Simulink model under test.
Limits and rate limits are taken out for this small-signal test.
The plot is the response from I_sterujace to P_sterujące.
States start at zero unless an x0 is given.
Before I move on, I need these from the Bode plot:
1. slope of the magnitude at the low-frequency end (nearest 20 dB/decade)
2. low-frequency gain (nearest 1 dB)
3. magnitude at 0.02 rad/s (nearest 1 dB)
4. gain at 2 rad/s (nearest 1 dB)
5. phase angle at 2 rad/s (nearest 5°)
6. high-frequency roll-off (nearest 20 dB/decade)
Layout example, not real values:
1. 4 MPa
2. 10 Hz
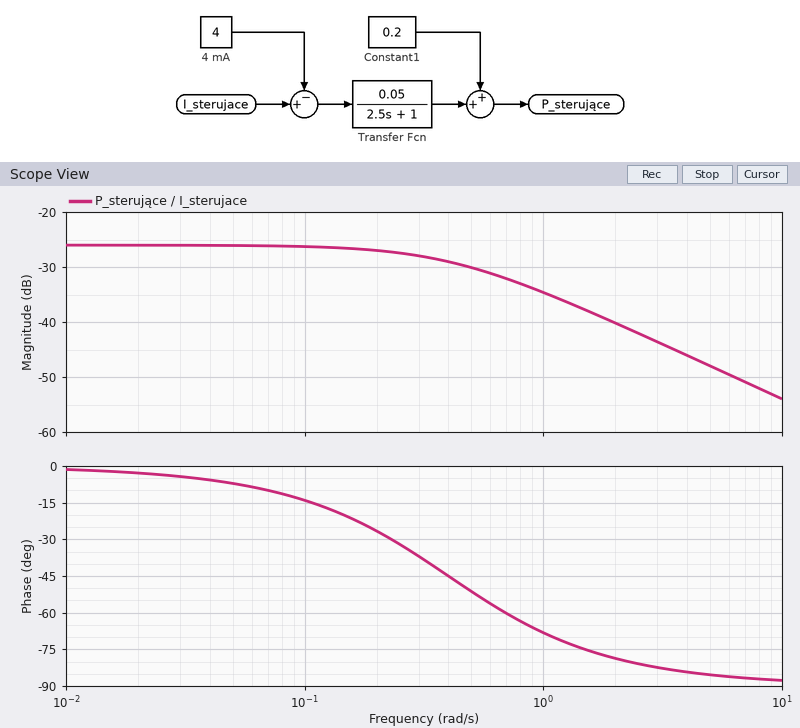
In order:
1. 0 dB/decade
2. -26 dB
3. -26 dB
4. -40 dB
5. -80°
6. -20 dB/decade
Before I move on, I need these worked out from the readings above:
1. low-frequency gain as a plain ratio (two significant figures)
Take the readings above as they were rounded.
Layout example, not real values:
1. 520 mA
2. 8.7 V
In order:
1. 0.050
